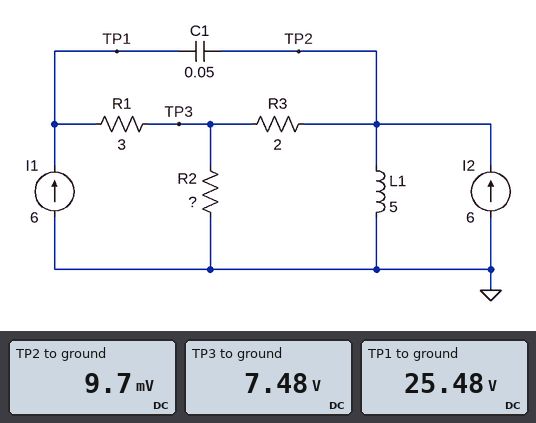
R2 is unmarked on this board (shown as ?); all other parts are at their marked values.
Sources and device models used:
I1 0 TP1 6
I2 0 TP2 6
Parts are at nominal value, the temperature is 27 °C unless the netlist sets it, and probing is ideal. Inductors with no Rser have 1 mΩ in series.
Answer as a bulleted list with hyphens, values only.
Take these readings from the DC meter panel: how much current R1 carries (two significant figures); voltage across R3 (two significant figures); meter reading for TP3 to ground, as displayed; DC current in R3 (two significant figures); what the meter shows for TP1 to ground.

- 6.0 A
- 7.5 V
- 7.48 V
- 3.7 A
- 25.48 V
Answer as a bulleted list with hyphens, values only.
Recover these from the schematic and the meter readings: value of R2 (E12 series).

- 3.3 Ω
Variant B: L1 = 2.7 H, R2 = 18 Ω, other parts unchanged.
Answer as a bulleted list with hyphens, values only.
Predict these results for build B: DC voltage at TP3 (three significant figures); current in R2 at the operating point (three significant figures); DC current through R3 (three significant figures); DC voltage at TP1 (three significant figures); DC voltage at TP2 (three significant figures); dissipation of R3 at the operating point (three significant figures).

- 10.8 V
- 601 mA
- 5.40 A
- 28.8 V
- 11.4 mV
- 58.3 W
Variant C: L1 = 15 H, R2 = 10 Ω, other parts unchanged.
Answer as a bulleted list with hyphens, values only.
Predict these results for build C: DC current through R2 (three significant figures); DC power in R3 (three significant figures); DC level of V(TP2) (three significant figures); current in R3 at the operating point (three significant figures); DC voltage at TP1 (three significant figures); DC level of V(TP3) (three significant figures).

- 1.00 A
- 50.0 W
- 11.0 mV
- 5.00 A
- 28.0 V
- 10.0 V
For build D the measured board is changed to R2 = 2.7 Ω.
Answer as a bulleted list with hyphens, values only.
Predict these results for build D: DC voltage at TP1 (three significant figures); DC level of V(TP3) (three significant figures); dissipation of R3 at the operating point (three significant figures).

- 24.9 V
- 6.90 V
- 23.7 W
